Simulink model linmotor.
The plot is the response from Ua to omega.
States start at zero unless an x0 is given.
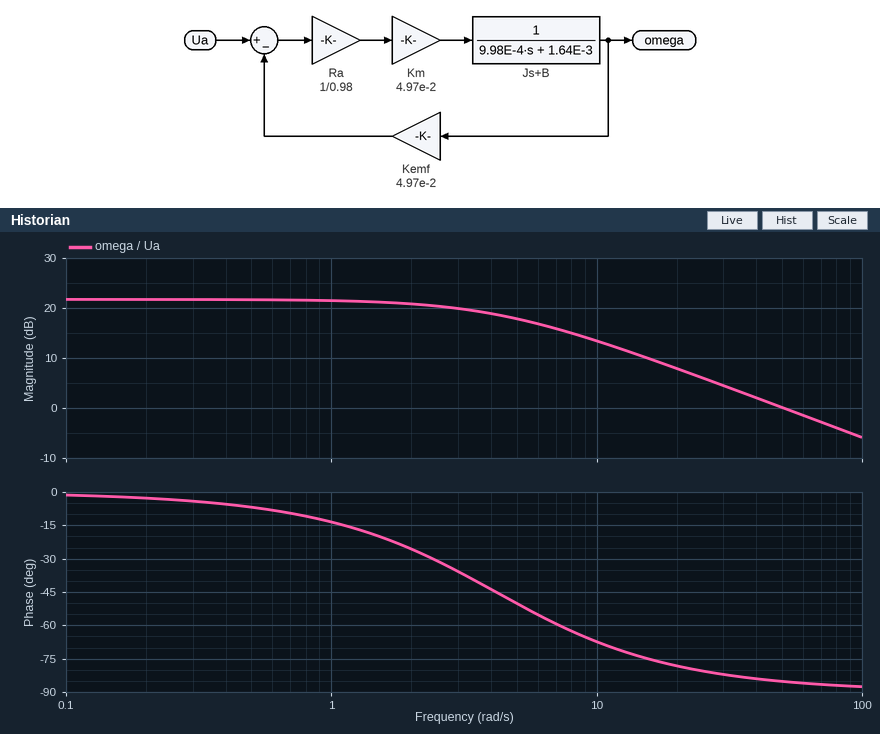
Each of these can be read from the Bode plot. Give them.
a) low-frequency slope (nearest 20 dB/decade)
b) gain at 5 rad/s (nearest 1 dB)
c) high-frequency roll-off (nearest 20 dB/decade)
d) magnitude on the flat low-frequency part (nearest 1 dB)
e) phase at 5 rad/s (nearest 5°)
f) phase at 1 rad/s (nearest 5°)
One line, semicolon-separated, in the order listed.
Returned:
0 dB/decade; 18 dB; -20 dB/decade; 22 dB; -50°; -15°
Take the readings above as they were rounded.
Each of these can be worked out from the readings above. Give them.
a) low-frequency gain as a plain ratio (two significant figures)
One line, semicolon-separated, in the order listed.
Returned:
13
